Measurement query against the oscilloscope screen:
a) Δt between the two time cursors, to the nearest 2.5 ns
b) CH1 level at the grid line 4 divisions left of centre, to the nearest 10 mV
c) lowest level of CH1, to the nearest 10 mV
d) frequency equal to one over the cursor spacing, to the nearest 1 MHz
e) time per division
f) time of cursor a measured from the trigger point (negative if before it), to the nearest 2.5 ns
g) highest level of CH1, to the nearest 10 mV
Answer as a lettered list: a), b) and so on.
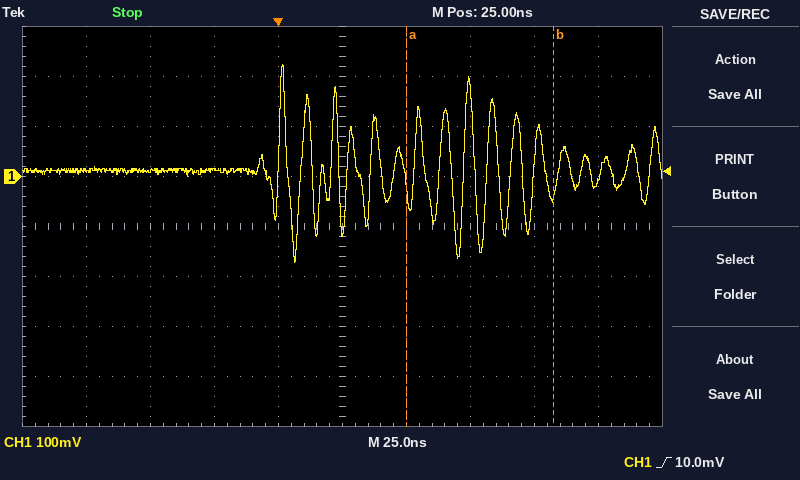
a) 57.5 ns
b) 10 mV
c) -170 mV
d) 17 MHz
e) 25 ns
f) +50.0 ns
g) 220 mV
